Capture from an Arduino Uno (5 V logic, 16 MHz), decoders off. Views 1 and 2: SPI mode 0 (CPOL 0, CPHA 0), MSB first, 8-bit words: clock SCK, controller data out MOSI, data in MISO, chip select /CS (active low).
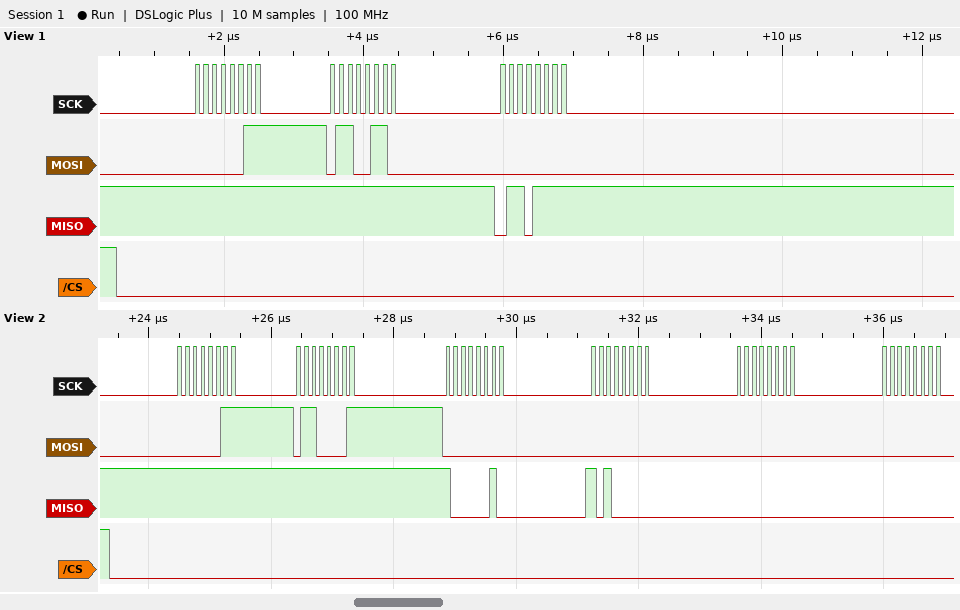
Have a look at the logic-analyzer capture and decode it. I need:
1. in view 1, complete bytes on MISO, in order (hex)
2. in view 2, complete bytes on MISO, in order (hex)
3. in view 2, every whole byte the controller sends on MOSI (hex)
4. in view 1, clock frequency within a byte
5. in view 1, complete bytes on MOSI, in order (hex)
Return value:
0xFF 0xFF 0x6F
FF FF 82 A0 00 00
03 61 00 00 00 00
8 MHz
0x03 0x66 0x00
